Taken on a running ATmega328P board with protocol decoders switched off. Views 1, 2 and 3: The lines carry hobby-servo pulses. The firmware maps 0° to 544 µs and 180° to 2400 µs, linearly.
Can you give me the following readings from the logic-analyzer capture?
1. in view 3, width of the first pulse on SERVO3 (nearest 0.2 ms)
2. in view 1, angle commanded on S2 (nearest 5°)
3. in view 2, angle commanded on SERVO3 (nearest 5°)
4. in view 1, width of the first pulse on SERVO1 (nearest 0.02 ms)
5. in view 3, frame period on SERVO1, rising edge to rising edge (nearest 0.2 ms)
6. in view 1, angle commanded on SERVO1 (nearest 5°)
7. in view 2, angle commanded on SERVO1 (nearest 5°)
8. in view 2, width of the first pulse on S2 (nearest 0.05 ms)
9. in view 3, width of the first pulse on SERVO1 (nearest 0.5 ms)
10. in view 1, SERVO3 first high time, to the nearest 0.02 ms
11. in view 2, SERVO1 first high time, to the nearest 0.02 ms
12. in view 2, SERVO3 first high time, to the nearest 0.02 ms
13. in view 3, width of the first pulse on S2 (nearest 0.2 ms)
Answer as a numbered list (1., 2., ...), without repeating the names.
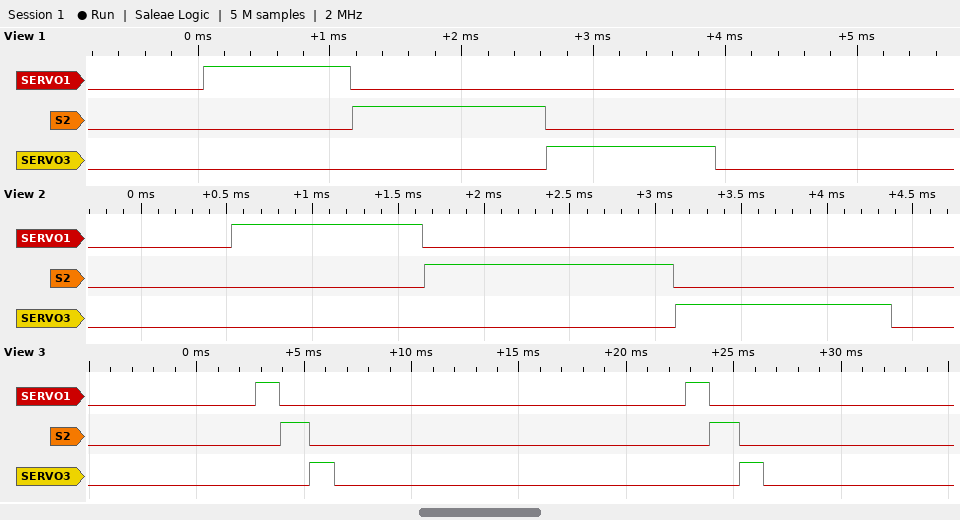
1. 1.2 ms
2. 90°
3. 70°
4. 1.12 ms
5. 20.0 ms
6. 55°
7. 55°
8. 1.45 ms
9. 1.0 ms
10. 1.28 ms
11. 1.12 ms
12. 1.26 ms
13. 1.4 ms
